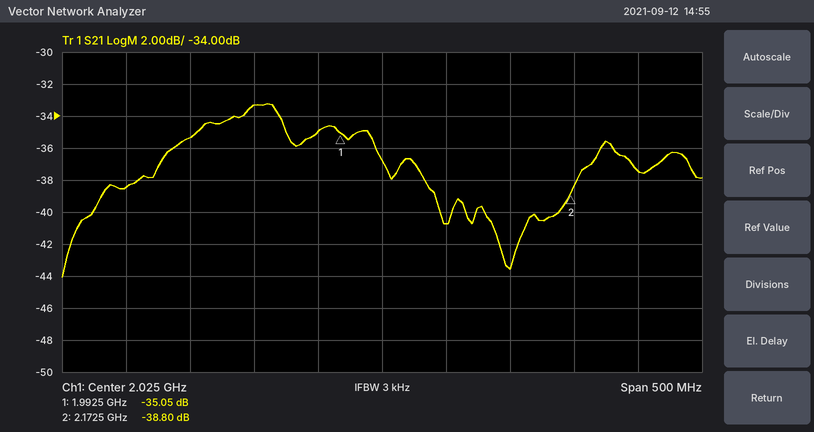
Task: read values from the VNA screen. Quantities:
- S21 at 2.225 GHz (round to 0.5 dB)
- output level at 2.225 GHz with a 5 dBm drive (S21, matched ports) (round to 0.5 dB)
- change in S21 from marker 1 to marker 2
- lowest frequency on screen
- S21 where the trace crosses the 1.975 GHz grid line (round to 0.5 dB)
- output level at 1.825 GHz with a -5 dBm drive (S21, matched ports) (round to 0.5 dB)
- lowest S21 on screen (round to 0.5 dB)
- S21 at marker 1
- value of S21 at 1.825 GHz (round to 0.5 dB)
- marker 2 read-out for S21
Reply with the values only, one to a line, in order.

-37.5 dB
-32.5 dBm
-3.75 dB
1.775 GHz
-35.0 dB
-43.5 dBm
-44.0 dB
-35.05 dB
-38.5 dB
-38.80 dB
